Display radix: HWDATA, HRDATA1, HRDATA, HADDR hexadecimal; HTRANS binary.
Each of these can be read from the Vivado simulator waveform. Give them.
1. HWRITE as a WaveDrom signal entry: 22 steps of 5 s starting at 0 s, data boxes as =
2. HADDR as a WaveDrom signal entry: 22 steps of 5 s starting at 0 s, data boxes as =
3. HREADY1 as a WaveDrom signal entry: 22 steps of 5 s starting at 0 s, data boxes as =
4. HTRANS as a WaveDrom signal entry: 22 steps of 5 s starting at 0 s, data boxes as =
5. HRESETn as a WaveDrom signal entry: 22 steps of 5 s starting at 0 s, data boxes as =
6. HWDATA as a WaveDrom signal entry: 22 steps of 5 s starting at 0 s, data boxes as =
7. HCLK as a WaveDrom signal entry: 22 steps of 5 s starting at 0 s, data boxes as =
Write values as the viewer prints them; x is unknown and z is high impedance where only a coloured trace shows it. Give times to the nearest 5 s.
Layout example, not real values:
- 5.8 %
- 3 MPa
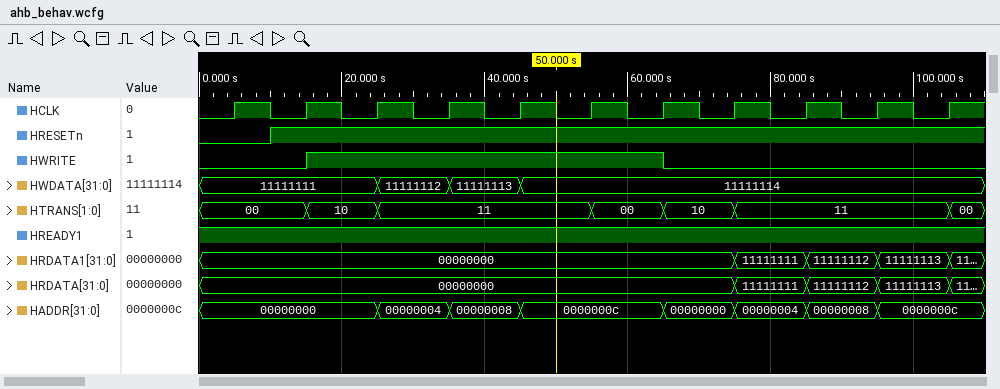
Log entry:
- {name: 'HWRITE', wave: '0..1.........0........'}
- {name: 'HADDR', wave: '=....=.=.=...=.=.=.=..', data: '00000000 00000004 00000008 0000000c 00000000 00000004 00000008 0000000c'}
- {name: 'HREADY1', wave: '1.....................'}
- {name: 'HTRANS', wave: '=..=.=.....=.=.=.....=', data: '00 10 11 00 10 11 00'}
- {name: 'HRESETn', wave: '0.1...................'}
- {name: 'HWDATA', wave: '=....=.=.=............', data: '11111111 11111112 11111113 11111114'}
- {name: 'HCLK', wave: '0101010101010101010101'}
